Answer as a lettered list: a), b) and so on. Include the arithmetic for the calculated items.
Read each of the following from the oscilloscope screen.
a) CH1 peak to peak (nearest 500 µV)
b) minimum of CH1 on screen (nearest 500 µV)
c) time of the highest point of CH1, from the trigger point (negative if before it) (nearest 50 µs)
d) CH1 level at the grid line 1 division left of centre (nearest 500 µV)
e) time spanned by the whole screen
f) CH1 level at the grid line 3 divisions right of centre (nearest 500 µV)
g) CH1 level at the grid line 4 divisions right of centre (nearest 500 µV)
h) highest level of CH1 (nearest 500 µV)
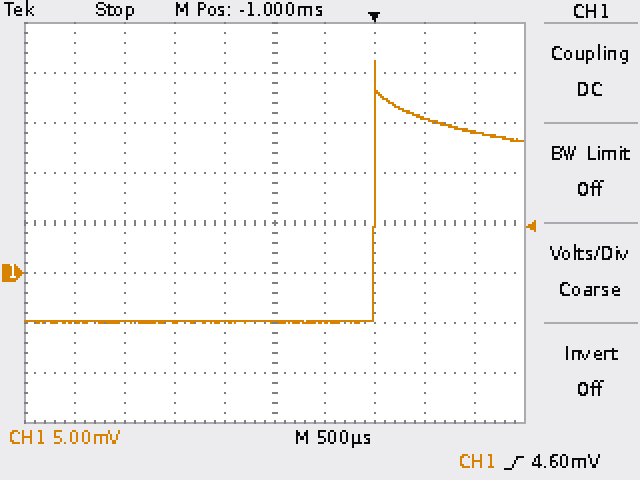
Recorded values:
a) 21.0 mV − (-5.0 mV) = 26.0 mV
b) -5.0 mV
c) 0 µs
d) -5.0 mV
e) 5 ms
f) 15.5 mV
g) 14.0 mV
h) 21.0 mV
